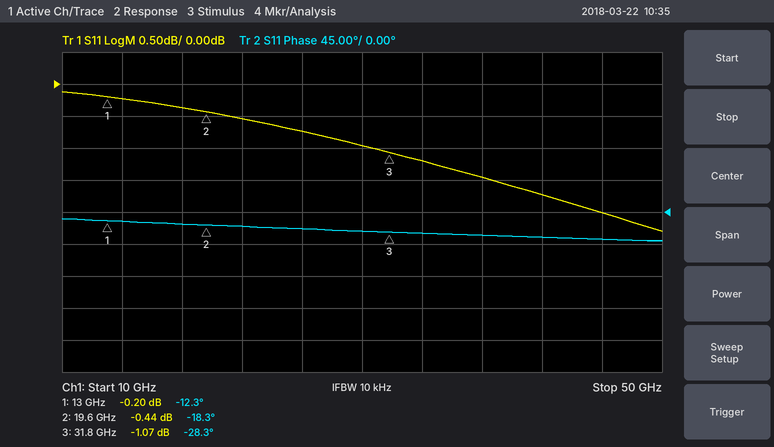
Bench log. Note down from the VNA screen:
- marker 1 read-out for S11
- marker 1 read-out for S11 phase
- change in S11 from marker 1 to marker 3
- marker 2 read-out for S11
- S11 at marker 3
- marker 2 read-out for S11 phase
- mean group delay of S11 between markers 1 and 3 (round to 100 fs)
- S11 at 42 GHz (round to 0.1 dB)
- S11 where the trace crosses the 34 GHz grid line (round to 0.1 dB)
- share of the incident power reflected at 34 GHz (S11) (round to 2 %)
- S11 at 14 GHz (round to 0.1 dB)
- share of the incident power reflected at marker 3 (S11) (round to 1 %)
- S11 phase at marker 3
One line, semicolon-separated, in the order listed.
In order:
-0.20 dB; -12.3°; -0.87 dB; -0.44 dB; -1.07 dB; -18.3°; 2.4 ps; -1.7 dB; -1.2 dB; 76 %; -0.2 dB; 78 %; -28.3°
